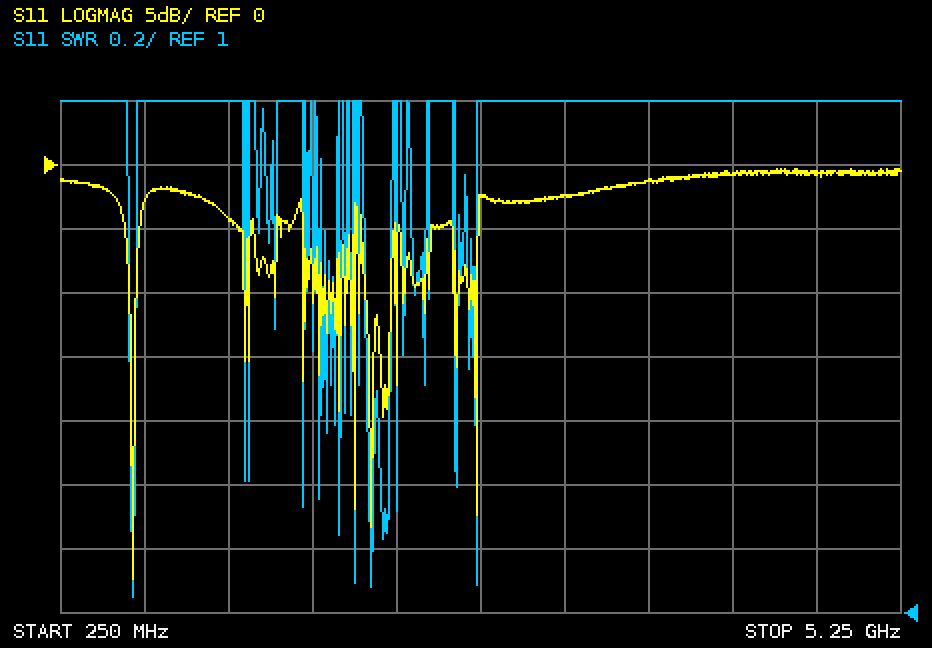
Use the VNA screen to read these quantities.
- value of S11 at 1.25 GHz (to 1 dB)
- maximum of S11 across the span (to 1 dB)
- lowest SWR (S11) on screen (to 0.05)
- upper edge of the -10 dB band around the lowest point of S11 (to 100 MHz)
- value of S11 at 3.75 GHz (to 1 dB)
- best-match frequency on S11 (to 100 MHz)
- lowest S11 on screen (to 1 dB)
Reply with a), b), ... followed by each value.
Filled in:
a) -4 dB
b) 0 dB
c) 1.05
d) 700 MHz
e) -1 dB
f) 700 MHz
g) -32 dB
